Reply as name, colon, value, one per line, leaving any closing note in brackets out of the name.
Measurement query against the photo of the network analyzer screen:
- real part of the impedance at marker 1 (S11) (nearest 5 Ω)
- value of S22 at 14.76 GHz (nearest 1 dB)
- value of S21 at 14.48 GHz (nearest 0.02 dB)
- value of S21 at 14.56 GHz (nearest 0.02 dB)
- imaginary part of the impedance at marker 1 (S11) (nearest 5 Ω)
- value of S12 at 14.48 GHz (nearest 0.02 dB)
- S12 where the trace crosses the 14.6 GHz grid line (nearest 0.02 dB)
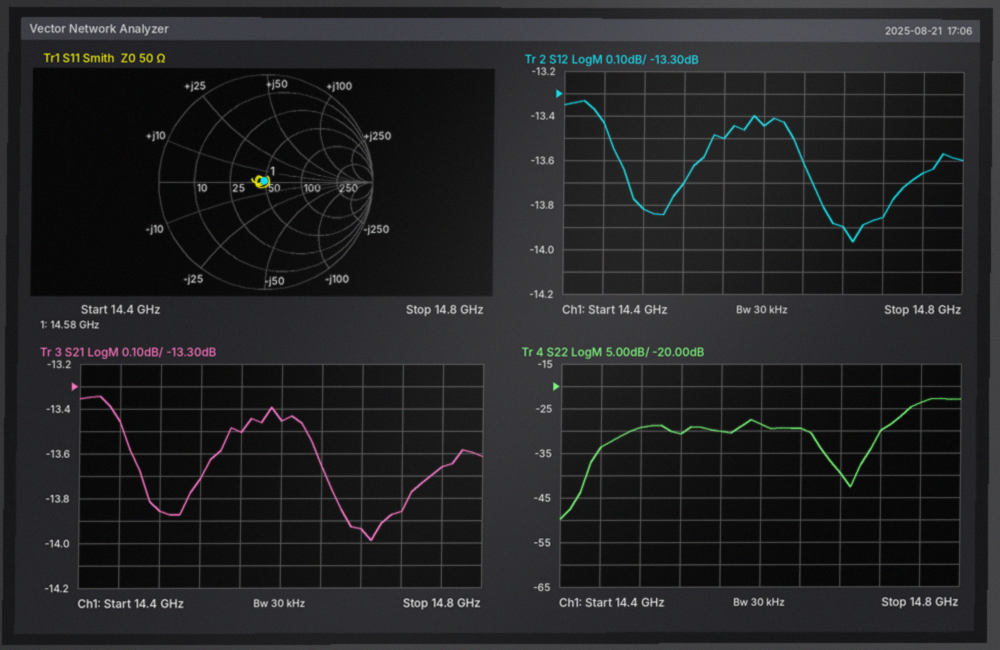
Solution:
real part of the impedance at marker 1 (S11): 50 Ω
value of S22 at 14.76 GHz: -24 dB
value of S21 at 14.48 GHz: -13.86 dB
value of S21 at 14.56 GHz: -13.50 dB
imaginary part of the impedance at marker 1 (S11): 0 Ω
value of S12 at 14.48 GHz: -13.82 dB
S12 where the trace crosses the 14.6 GHz grid line: -13.44 dB
